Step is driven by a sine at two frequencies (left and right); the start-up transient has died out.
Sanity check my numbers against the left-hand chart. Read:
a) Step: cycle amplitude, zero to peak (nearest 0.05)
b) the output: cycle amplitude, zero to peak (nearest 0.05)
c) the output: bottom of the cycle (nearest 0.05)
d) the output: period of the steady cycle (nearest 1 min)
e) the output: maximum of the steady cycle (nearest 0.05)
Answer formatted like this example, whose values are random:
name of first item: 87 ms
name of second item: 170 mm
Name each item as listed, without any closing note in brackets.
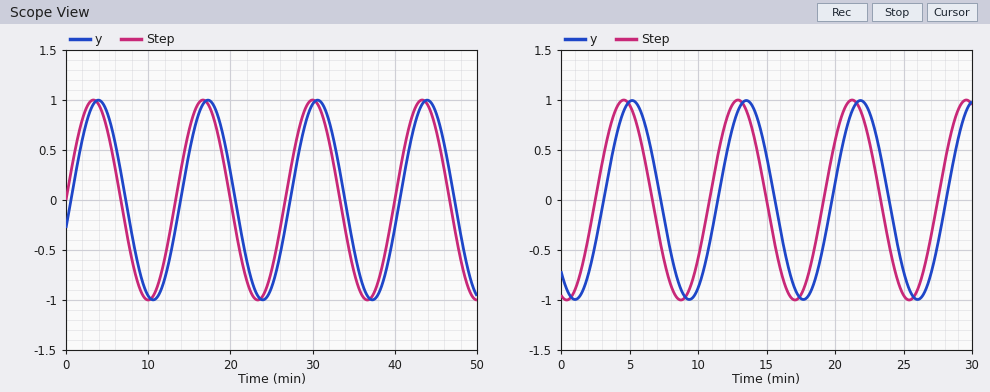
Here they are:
Step: cycle amplitude, zero to peak: 1.00
the output: cycle amplitude, zero to peak: 1.00
the output: bottom of the cycle: -1.00
the output: period of the steady cycle: 13 min
the output: maximum of the steady cycle: 1.00
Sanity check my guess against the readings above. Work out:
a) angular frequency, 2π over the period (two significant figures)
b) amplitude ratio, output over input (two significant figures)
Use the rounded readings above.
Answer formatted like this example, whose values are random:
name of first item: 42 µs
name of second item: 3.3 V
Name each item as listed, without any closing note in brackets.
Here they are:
angular frequency, 2π over the period: 0.48 rad/min
amplitude ratio, output over input: 1.0
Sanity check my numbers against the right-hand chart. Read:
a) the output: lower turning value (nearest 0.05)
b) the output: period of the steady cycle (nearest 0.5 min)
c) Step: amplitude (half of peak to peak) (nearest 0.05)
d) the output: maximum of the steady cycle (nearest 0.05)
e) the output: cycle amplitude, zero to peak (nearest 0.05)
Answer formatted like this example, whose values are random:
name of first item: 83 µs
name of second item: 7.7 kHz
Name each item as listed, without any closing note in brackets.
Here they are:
the output: lower turning value: -1.00
the output: period of the steady cycle: 8.5 min
Step: amplitude (half of peak to peak): 1.00
the output: maximum of the steady cycle: 1.00
the output: cycle amplitude, zero to peak: 1.00
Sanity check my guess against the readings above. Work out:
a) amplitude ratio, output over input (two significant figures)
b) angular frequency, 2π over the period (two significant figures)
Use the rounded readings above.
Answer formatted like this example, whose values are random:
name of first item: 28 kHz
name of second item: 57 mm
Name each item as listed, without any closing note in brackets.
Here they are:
amplitude ratio, output over input: 1.0
angular frequency, 2π over the period: 0.74 rad/min
